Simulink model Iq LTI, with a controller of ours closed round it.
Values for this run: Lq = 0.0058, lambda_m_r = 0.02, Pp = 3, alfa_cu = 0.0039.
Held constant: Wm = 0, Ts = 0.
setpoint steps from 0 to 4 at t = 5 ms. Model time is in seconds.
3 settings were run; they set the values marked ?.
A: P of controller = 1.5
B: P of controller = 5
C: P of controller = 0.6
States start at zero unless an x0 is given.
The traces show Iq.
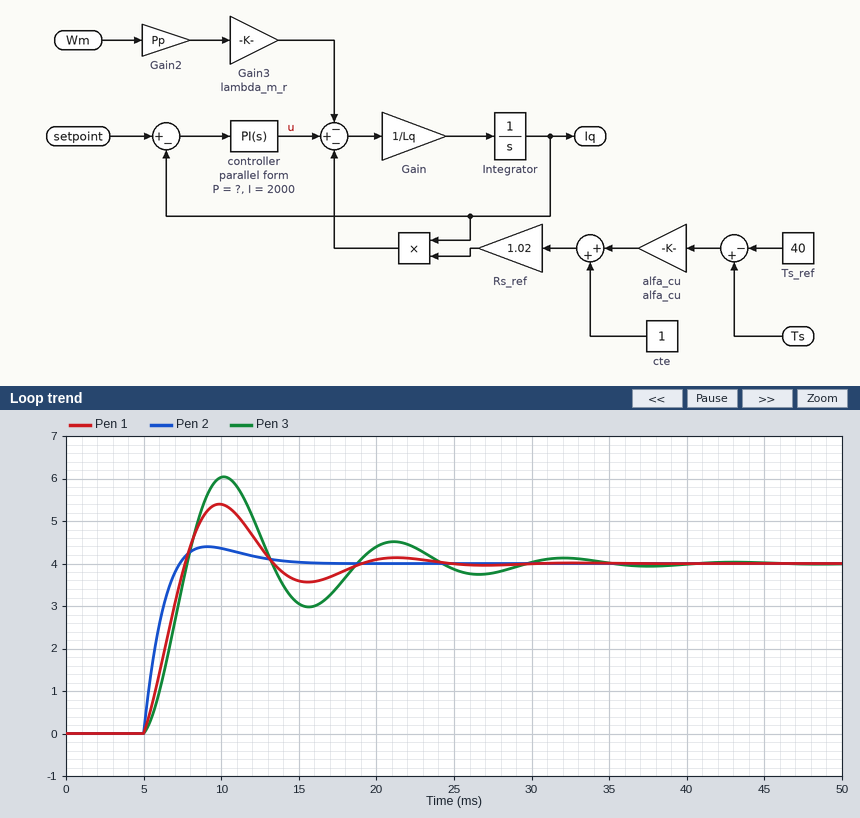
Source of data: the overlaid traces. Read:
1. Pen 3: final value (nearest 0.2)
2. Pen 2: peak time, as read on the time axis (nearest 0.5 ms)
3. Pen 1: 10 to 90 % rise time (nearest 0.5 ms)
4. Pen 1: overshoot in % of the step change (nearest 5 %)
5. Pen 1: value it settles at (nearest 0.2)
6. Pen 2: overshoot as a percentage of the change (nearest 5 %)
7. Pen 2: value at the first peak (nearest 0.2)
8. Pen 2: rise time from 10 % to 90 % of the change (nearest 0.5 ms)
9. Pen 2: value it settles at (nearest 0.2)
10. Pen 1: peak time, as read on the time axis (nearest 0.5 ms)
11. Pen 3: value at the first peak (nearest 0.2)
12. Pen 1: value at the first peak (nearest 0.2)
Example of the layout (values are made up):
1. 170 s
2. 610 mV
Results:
1. 4.0
2. 9.0 ms
3. 2.0 ms
4. 35 %
5. 4.0
6. 10 %
7. 4.4
8. 1.5 ms
9. 4.0
10. 10.0 ms
11. 6.0
12. 5.4
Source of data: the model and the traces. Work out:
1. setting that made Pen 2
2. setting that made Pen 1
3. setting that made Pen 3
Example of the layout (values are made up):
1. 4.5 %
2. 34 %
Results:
1. B
2. A
3. C
